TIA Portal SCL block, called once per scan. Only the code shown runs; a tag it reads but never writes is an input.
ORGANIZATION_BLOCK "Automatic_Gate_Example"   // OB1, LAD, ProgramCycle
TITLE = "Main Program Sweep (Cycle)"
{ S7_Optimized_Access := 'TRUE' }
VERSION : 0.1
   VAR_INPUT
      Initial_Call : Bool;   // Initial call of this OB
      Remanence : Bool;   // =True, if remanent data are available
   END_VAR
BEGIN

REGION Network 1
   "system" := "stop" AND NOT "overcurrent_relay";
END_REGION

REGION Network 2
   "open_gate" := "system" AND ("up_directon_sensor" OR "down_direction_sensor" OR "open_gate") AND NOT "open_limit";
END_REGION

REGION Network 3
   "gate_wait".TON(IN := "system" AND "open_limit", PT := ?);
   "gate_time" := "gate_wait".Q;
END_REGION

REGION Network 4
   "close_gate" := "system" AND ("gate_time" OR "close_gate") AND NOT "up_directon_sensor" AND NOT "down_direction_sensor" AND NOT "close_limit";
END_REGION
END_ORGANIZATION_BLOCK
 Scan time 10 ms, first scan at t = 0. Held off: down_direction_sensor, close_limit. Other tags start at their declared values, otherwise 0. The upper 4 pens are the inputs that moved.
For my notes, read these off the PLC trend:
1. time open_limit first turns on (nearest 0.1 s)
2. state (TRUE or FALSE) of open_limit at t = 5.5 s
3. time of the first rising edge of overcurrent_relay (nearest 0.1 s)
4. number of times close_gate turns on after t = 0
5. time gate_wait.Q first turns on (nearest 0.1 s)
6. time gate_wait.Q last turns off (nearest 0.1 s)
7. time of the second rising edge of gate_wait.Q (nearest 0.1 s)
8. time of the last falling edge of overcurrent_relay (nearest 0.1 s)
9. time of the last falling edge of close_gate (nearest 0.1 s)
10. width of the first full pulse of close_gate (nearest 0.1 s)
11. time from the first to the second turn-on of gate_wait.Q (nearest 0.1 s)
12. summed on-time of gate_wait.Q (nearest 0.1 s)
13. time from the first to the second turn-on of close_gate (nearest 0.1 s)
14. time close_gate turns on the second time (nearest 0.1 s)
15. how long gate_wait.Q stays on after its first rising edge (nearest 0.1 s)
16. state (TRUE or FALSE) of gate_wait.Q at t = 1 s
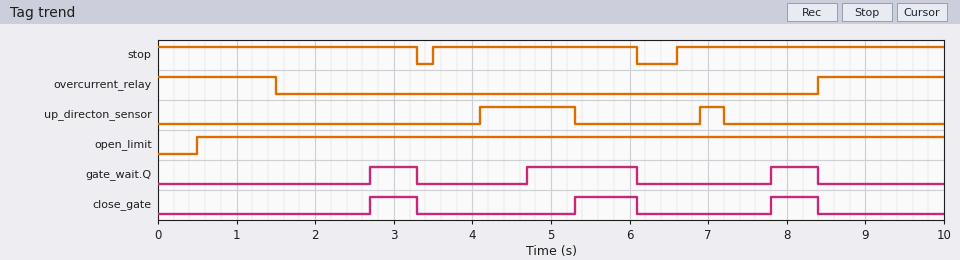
0.5 s
TRUE
8.4 s
3
2.7 s
8.4 s
4.7 s
1.5 s
8.4 s
0.6 s
2.0 s
2.6 s
2.6 s
5.3 s
0.6 s
FALSE
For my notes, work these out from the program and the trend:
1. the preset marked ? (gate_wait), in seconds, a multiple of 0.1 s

1.2 s
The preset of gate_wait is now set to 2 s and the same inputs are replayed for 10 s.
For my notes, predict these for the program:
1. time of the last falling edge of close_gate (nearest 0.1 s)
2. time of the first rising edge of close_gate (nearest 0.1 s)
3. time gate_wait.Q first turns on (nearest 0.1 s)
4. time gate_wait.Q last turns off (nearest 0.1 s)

6.1 s
5.5 s
5.5 s
6.1 s
